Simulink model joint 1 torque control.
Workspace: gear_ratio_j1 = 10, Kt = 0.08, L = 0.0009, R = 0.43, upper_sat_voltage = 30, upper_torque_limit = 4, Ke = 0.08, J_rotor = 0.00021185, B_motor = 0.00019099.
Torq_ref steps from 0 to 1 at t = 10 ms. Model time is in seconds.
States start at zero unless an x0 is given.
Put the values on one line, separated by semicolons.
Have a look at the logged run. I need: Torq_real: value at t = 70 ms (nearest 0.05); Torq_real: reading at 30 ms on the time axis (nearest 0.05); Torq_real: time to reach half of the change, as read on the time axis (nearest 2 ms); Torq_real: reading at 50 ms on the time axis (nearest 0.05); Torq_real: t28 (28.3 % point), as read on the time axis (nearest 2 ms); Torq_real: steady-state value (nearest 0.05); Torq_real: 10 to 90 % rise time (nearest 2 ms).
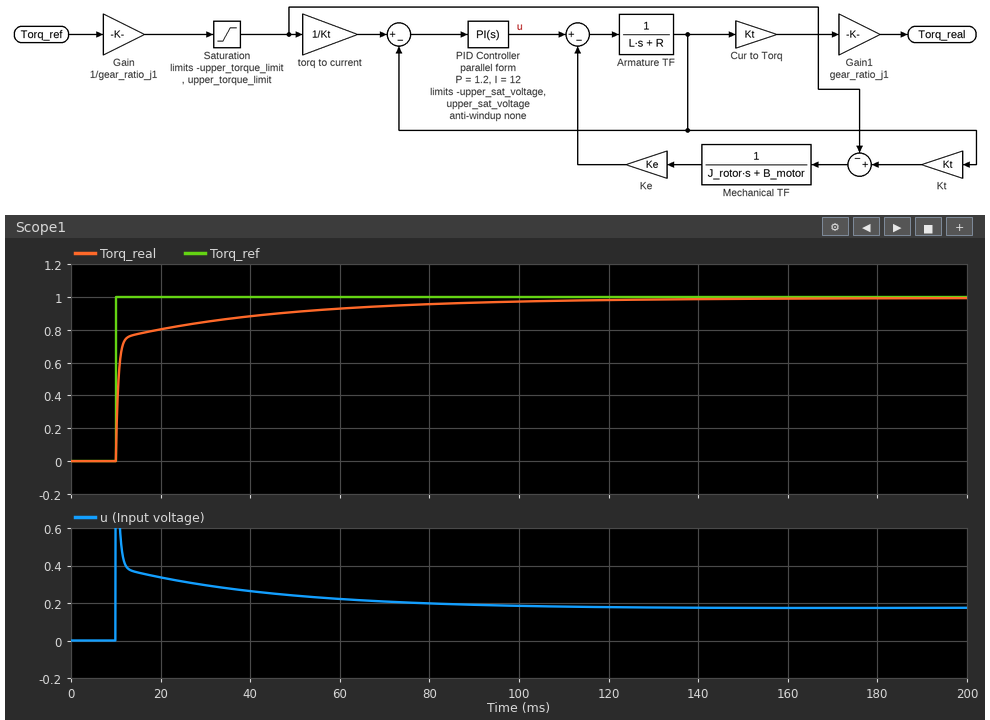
0.95; 0.85; 10 ms; 0.90; 10 ms; 1.00; 34 ms
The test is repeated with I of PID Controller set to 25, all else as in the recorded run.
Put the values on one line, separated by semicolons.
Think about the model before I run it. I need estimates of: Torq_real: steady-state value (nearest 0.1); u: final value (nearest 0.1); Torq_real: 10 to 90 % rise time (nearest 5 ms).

1.0; 0.3; 25 ms
